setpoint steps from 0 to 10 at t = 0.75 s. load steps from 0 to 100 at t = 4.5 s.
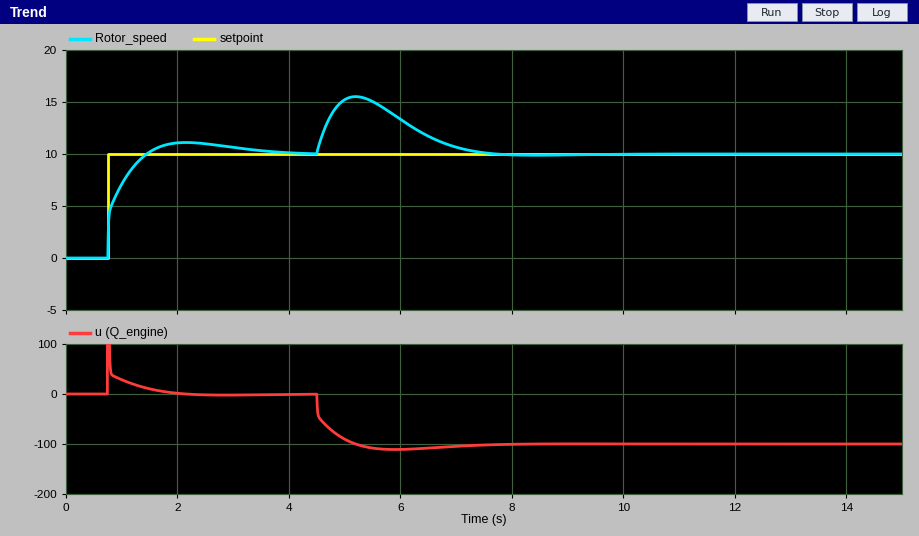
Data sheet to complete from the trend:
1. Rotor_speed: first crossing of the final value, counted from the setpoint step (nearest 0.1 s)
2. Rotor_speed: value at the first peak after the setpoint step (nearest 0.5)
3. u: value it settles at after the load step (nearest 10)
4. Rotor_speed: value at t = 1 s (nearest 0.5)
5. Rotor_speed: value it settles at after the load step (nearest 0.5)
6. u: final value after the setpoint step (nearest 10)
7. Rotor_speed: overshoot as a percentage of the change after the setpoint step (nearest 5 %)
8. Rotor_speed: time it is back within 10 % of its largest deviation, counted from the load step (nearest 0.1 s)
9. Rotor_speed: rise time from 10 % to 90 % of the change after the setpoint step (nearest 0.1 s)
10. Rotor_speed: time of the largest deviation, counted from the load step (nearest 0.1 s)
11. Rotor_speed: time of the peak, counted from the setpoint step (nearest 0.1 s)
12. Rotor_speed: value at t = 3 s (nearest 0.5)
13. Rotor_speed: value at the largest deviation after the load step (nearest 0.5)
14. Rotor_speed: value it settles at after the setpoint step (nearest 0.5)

0.7 s
11.0
-100
7.0
10.0
0
10 %
2.6 s
0.5 s
0.7 s
1.4 s
10.5
15.5
10.0
